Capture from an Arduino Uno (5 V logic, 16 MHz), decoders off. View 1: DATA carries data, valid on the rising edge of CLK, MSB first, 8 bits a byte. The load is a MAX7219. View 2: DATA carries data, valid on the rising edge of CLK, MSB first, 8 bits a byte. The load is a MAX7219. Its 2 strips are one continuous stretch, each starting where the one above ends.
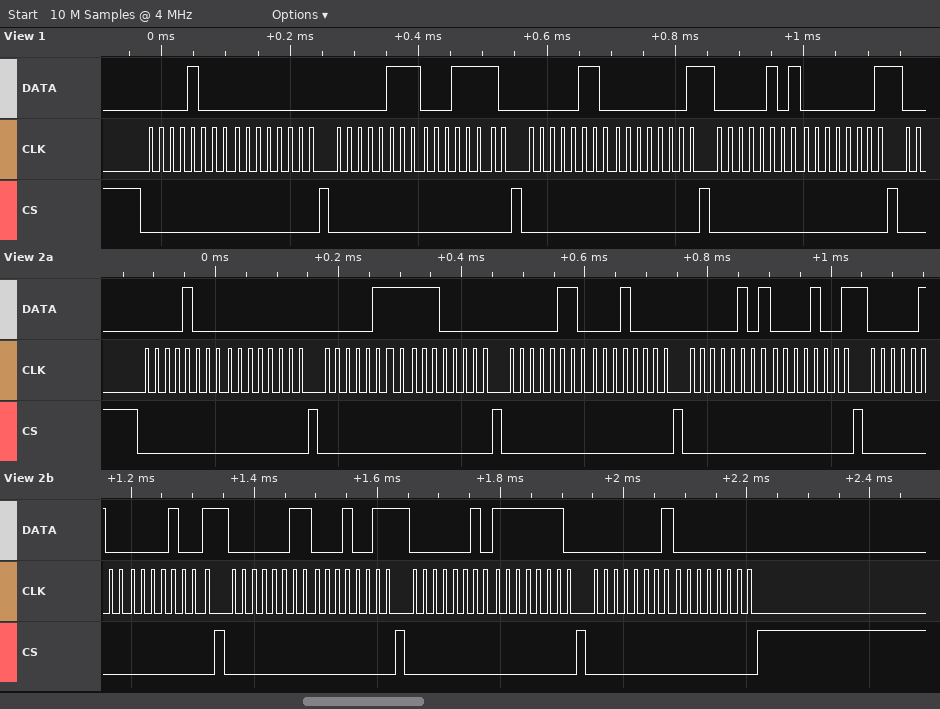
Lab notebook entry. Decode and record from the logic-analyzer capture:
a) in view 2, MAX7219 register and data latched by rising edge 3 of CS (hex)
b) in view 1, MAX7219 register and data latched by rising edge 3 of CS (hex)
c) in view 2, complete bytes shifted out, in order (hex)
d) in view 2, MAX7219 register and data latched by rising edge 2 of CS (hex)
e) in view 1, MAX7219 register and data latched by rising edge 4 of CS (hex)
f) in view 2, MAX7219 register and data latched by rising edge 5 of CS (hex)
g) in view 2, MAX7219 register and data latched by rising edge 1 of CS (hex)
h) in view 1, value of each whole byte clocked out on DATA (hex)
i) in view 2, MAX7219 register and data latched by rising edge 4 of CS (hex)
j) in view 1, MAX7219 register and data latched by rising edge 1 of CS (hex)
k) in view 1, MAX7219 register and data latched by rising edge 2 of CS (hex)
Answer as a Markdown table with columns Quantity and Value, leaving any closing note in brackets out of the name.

| Quantity | Value |
|---|---|
| in view 2, MAX7219 register and data latched by rising edge 3 of CS | register 0x6, data 0x10 |
| in view 1, MAX7219 register and data latched by rising edge 3 of CS | register 0x6, data 0x01 |
| in view 2, complete bytes shifted out, in order | 0x08 0x00 0x07 0xE0 0x06 0x10 0x05 0x09 0x04 0x09 0x03 0x13 0x02 0xFE 0x01 0x00 |
| in view 2, MAX7219 register and data latched by rising edge 2 of CS | register 0x7, data 0xE0 |
| in view 1, MAX7219 register and data latched by rising edge 4 of CS | register 0x5, data 0x01 |
| in view 2, MAX7219 register and data latched by rising edge 5 of CS | register 0x4, data 0x09 |
| in view 2, MAX7219 register and data latched by rising edge 1 of CS | register 0x8, data 0x00 |
| in view 1, value of each whole byte clocked out on DATA | 0x08 0x00 0x07 0x1E 0x06 0x01 0x05 0x01 |
| in view 2, MAX7219 register and data latched by rising edge 4 of CS | register 0x5, data 0x09 |
| in view 1, MAX7219 register and data latched by rising edge 1 of CS | register 0x8, data 0x00 |
| in view 1, MAX7219 register and data latched by rising edge 2 of CS | register 0x7, data 0x1E |
